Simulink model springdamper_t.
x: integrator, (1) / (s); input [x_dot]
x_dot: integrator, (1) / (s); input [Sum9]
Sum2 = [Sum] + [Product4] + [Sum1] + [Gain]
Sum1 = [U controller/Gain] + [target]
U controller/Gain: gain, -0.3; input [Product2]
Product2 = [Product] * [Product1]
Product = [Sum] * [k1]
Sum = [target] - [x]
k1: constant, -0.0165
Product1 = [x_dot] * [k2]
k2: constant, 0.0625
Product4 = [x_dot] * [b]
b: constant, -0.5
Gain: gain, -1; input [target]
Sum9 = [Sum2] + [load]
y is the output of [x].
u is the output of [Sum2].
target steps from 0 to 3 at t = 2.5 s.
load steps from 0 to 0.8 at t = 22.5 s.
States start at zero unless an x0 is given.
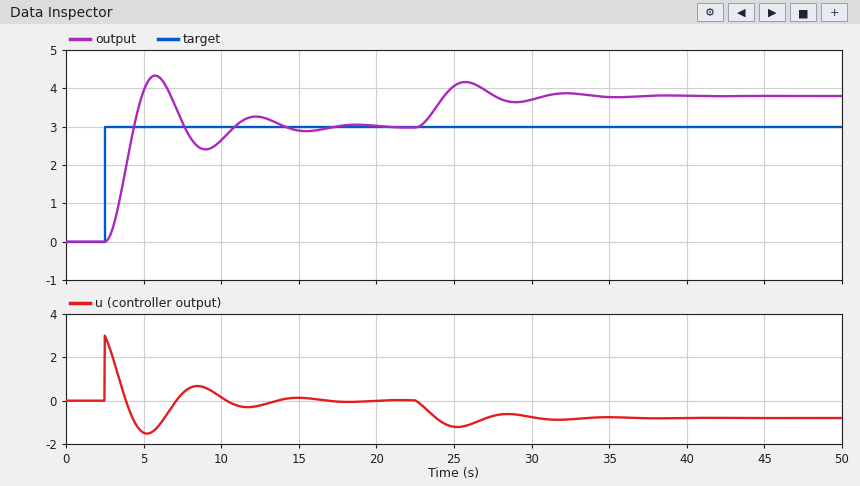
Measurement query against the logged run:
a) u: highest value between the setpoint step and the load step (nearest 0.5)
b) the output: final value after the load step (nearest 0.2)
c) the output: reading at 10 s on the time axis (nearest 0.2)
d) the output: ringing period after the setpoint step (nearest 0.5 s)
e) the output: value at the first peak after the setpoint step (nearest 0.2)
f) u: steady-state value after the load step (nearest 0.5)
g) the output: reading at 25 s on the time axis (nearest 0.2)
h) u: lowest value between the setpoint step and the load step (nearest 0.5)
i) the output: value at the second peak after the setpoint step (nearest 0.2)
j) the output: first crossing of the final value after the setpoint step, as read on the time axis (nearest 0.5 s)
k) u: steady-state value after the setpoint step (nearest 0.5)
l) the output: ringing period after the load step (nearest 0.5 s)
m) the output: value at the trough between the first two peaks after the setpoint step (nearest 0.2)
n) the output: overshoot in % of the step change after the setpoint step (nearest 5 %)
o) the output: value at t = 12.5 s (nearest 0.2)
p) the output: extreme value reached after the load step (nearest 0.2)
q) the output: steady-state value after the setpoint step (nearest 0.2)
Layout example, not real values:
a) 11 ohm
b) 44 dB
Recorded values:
a) 3.0
b) 3.8
c) 2.6
d) 6.5 s
e) 4.4
f) -1.0
g) 4.0
h) -1.5
i) 3.2
j) 4.5 s
k) 0.0
l) 6.5 s
m) 2.4
n) 45 %
o) 3.2
p) 4.2
q) 3.0
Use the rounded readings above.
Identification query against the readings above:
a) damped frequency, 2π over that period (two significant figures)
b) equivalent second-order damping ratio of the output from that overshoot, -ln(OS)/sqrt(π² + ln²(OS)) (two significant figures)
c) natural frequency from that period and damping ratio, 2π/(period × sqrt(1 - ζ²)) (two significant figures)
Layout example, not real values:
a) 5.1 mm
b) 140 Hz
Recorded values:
a) 0.97 rad/s
b) 0.25
c) 1.00 rad/s
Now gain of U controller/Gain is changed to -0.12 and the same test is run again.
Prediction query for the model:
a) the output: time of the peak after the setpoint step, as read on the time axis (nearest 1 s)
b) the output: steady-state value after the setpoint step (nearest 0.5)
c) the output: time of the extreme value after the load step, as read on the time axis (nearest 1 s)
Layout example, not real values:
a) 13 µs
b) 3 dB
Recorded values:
a) 6 s
b) 3.0
c) 26 s
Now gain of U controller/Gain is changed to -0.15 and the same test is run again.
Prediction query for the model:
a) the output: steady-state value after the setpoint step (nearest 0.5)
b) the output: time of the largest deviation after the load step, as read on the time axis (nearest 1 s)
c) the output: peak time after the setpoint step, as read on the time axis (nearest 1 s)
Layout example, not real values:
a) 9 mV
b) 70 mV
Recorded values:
a) 3.0
b) 26 s
c) 6 s
